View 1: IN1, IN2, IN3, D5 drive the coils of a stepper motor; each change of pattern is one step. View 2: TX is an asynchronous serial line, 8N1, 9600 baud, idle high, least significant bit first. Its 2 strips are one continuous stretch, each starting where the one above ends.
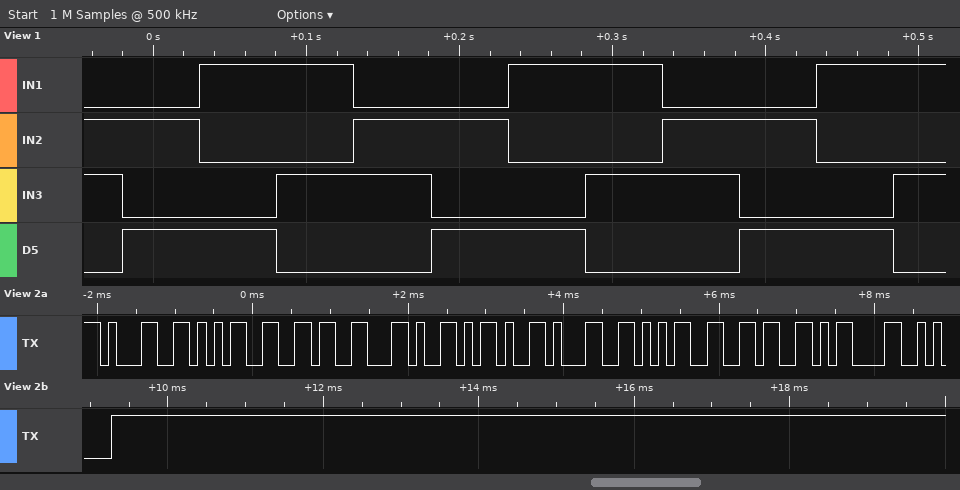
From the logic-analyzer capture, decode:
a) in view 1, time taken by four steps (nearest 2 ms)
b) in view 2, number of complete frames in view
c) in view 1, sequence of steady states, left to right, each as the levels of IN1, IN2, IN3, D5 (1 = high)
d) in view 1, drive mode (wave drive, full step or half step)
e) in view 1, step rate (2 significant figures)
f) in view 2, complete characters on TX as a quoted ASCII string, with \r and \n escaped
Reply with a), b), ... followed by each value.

a) 202 ms
b) 10
c) 0110 0101 1001 1010 0110 0101 1001 1010 0110 0101 1001 1010
d) full step
e) 20 steps/s
f) "156,-156\r\n"
